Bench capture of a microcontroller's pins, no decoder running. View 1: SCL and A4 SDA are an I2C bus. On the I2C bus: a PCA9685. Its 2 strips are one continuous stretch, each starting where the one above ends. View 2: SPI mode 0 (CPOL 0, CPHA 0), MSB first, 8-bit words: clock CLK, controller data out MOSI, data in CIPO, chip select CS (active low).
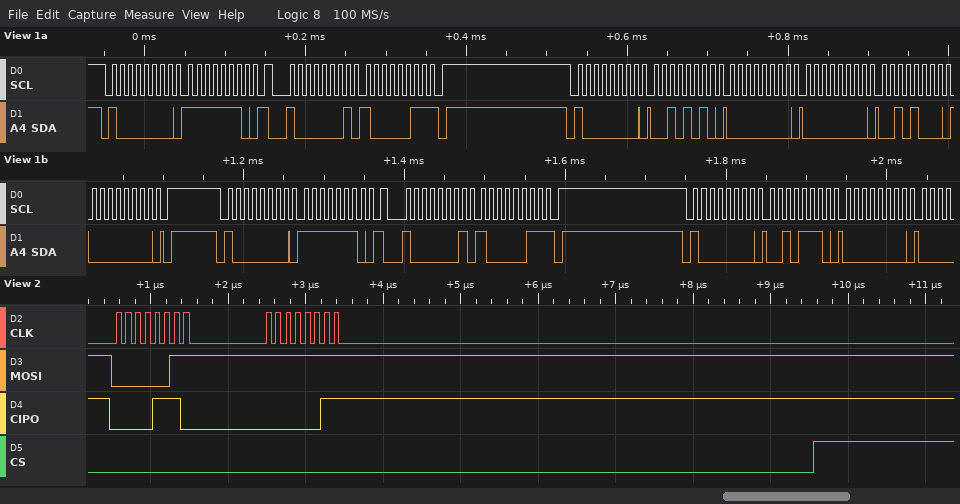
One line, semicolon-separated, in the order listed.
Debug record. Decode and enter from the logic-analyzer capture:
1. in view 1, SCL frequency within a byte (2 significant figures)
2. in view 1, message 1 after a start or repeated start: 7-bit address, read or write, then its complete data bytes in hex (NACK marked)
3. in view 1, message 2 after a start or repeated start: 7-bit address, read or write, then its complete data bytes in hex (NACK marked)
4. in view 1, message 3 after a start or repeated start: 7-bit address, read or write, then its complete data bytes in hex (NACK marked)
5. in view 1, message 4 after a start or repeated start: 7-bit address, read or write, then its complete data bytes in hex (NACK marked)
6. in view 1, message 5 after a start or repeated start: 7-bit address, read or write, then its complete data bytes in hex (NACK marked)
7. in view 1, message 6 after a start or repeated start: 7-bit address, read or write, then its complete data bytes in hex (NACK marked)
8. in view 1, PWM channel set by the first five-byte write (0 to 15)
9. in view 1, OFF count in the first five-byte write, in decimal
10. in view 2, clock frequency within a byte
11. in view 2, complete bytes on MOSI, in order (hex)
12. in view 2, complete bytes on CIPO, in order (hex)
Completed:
100 kHz; 0x40 write: FE; 0x40 read: 83 NACK; 0x40 write: 2A 00 00 28 00; 0x40 write: FE; 0x40 read: 83 NACK; 0x40 write: 2E 00; 9; 40; 8 MHz; 03 FF; 0E 03
